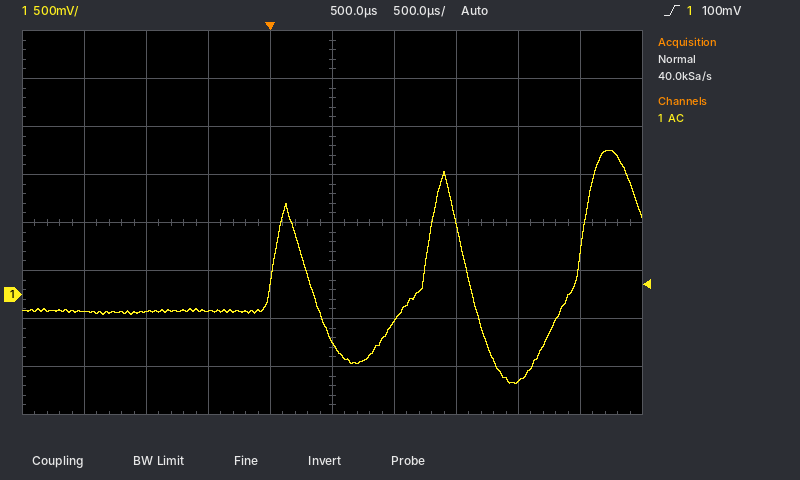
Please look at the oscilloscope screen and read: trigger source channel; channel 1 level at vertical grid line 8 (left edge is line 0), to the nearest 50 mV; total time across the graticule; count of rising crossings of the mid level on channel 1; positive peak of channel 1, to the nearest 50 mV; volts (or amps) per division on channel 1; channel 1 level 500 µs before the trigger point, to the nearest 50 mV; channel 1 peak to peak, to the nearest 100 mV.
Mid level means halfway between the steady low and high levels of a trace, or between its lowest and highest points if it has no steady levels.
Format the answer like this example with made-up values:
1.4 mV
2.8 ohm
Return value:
channel 1
-900 mV
5 ms
3
1.50 V
500 mV
-150 mV
2.40 V
